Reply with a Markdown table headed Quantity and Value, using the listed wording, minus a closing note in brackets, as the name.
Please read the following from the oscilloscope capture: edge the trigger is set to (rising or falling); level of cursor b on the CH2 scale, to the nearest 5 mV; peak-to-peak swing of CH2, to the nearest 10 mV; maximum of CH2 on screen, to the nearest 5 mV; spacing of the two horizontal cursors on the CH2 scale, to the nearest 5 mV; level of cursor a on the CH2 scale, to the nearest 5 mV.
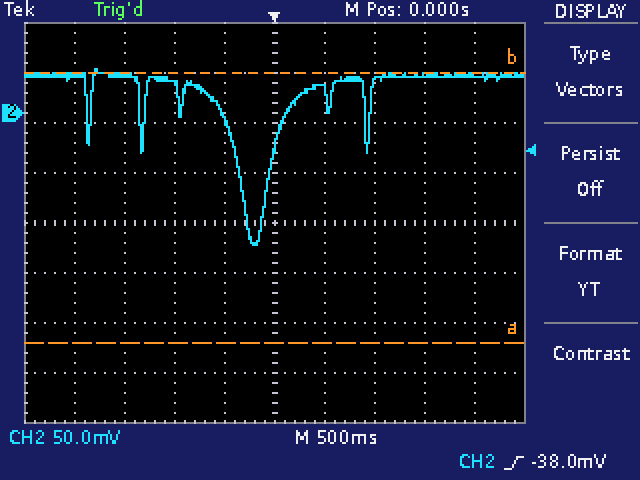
| Quantity | Value |
|---|---|
| edge the trigger is set to | rising |
| level of cursor b on the CH2 scale, to the nearest 5 mV | 40 mV |
| peak-to-peak swing of CH2, to the nearest 10 mV | 180 mV |
| maximum of CH2 on screen, to the nearest 5 mV | 45 mV |
| spacing of the two horizontal cursors on the CH2 scale, to the nearest 5 mV | 270 mV |
| level of cursor a on the CH2 scale, to the nearest 5 mV | -230 mV |
